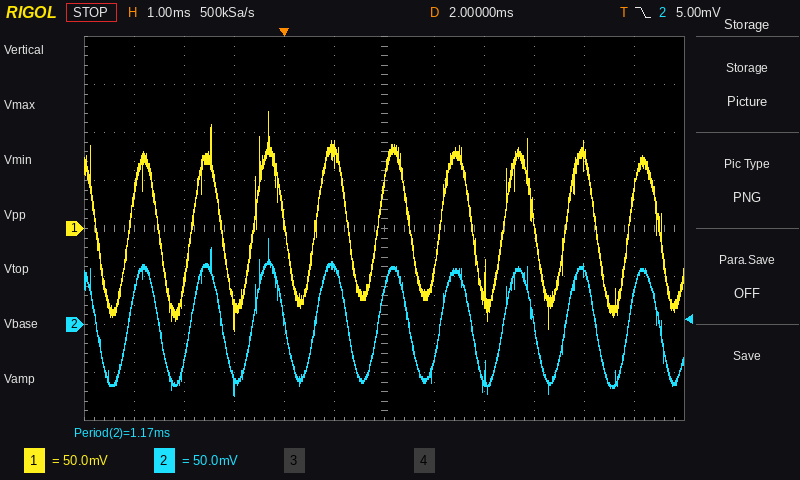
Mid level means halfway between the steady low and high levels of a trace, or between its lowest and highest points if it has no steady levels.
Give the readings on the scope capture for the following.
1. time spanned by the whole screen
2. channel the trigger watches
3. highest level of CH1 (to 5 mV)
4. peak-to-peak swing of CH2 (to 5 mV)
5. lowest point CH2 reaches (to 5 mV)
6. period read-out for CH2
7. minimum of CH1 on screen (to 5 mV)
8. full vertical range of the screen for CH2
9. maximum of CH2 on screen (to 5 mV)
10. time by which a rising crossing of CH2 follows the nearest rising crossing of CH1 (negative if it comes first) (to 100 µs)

12 ms
CH2
120 mV
165 mV
-75 mV
1.17 ms
-105 mV
400 mV
90 mV
0.0 ms
